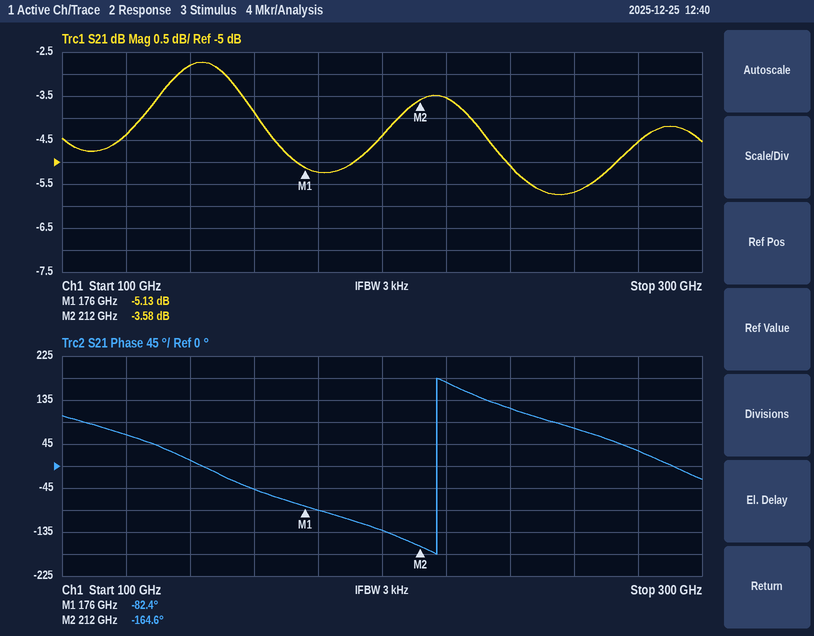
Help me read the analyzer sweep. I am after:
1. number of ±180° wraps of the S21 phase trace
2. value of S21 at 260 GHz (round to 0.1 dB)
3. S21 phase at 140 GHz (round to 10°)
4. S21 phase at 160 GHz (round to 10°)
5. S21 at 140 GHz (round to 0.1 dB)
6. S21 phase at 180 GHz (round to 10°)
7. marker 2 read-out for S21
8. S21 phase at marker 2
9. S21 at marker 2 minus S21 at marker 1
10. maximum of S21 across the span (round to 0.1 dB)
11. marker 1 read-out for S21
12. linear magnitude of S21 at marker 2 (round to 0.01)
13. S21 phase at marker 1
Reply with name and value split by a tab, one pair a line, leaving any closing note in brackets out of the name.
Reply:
number of ±180° wraps of the S21 phase trace	1
value of S21 at 260 GHz	-5.7 dB
S21 phase at 140 GHz	10°
S21 phase at 160 GHz	-50°
S21 at 140 GHz	-2.8 dB
S21 phase at 180 GHz	-90°
marker 2 read-out for S21	-3.58 dB
S21 phase at marker 2	-164.6°
S21 at marker 2 minus S21 at marker 1	1.55 dB
maximum of S21 across the span	-2.7 dB
marker 1 read-out for S21	-5.13 dB
linear magnitude of S21 at marker 2	0.66
S21 phase at marker 1	-82.4°
